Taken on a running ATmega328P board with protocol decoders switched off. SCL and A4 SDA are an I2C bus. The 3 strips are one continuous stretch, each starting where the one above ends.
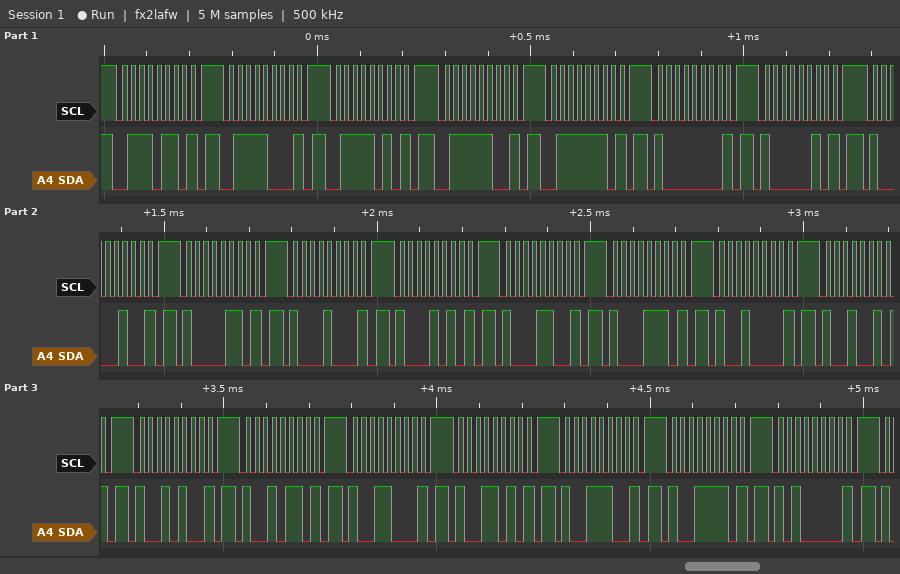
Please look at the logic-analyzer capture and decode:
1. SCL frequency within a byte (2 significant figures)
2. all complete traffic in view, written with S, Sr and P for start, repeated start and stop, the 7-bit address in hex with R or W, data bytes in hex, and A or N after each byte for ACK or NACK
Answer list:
50 kHz
S 3BW N P S 3CW N P S 3DW N P S 3EW N P S 3FW N P S 40W N P S 41W N P S 42W N P S 43W N P S 44W N P S 45W N P S 46W N P S 47W N P S 48W N P S 49W N P S 4AW N P S 4BW N P S 4CW N P S 4DW N P S 4EW N P S 4FW N P S 50W N P
